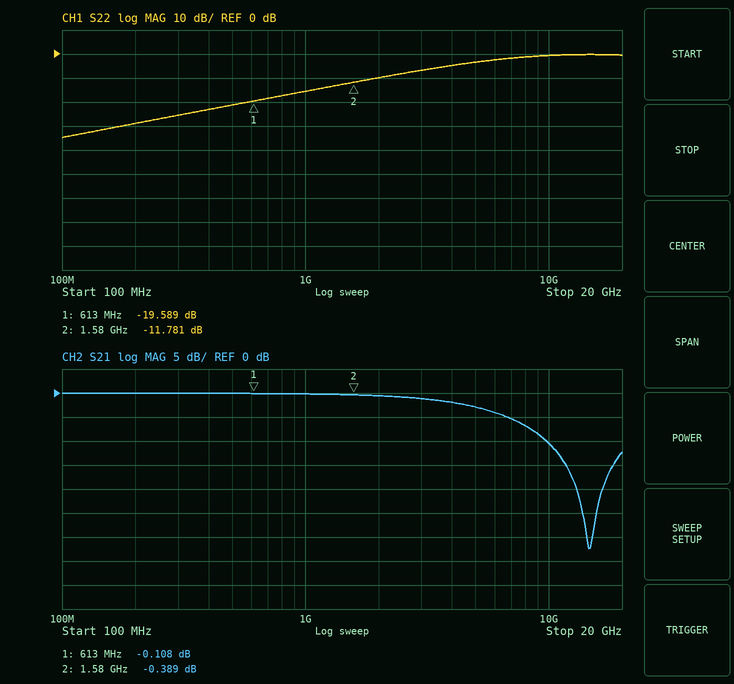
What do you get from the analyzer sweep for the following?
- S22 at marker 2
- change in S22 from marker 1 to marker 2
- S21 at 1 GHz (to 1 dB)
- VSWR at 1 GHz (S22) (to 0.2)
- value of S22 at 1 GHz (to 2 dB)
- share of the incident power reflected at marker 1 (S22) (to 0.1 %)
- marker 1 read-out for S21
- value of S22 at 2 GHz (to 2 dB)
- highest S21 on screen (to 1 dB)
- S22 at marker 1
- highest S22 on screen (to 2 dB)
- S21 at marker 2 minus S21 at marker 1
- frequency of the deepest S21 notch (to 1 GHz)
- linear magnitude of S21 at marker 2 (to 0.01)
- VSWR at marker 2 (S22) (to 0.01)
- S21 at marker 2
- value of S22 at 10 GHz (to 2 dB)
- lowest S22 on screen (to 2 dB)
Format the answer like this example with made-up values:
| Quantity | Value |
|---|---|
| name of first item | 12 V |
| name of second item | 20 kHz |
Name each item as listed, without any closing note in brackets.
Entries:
| Quantity | Value |
|---|---|
| S22 at marker 2 | -11.781 dB |
| change in S22 from marker 1 to marker 2 | 7.808 dB |
| S21 at 1 GHz | 0 dB |
| VSWR at 1 GHz (S22) | 1.4 |
| value of S22 at 1 GHz | -16 dB |
| share of the incident power reflected at marker 1 (S22) | 1.1 % |
| marker 1 read-out for S21 | -0.108 dB |
| value of S22 at 2 GHz | -10 dB |
| highest S21 on screen | 0 dB |
| S22 at marker 1 | -19.589 dB |
| highest S22 on screen | 0 dB |
| S21 at marker 2 minus S21 at marker 1 | -0.281 dB |
| frequency of the deepest S21 notch | 15 GHz |
| linear magnitude of S21 at marker 2 | 0.96 |
| VSWR at marker 2 (S22) | 1.69 |
| S21 at marker 2 | -0.389 dB |
| value of S22 at 10 GHz | 0 dB |
| lowest S22 on screen | -34 dB |
